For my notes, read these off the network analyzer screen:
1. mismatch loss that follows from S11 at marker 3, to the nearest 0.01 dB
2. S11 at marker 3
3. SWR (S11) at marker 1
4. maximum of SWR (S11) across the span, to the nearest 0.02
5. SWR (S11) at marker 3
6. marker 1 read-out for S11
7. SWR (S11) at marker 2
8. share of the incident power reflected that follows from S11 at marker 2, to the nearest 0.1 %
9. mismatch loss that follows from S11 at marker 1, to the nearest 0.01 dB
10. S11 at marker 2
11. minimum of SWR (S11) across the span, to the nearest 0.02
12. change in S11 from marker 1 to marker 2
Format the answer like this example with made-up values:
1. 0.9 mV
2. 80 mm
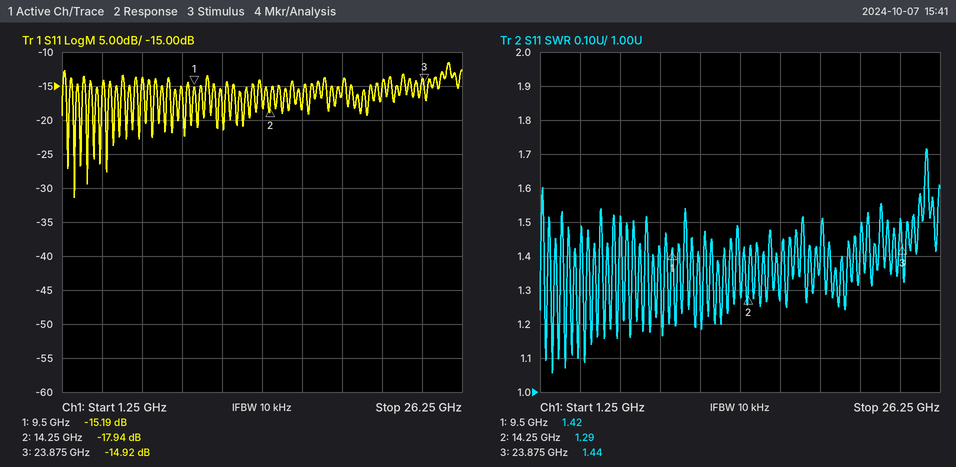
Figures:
1. 0.14 dB
2. -14.92 dB
3. 1.42
4. 1.72
5. 1.44
6. -15.19 dB
7. 1.29
8. 1.6 %
9. 0.13 dB
10. -17.94 dB
11. 1.06
12. -2.75 dB
